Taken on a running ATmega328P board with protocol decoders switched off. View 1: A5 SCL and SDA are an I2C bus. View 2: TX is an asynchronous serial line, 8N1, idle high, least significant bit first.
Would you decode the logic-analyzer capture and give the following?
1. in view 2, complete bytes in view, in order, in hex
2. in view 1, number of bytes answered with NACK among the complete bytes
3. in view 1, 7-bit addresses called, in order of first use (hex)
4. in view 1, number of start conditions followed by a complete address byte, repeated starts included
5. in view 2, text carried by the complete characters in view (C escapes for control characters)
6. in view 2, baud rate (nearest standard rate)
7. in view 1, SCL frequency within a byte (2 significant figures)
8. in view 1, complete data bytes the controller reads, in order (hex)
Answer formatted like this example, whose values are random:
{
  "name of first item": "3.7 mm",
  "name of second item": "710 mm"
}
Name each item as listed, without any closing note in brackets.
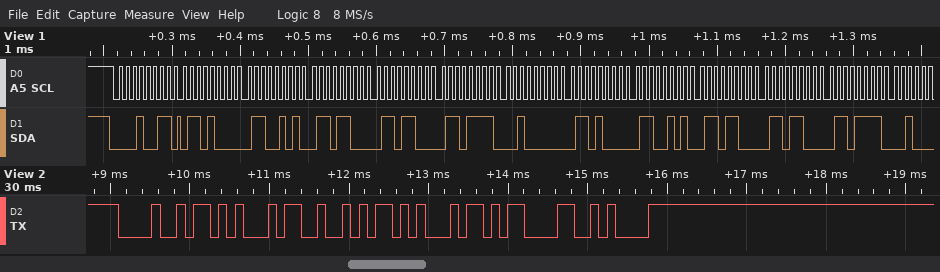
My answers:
{
  "in view 2, complete bytes in view, in order, in hex": "48 45 52 45 0D 0A",
  "in view 1, number of bytes answered with NACK among the complete bytes": "0",
  "in view 1, 7-bit addresses called, in order of first use": "0x09",
  "in view 1, number of start conditions followed by a complete address byte, repeated starts included": "1",
  "in view 2, text carried by the complete characters in view": "\"HERE\\r\\n\"",
  "in view 2, baud rate": "9600 baud",
  "in view 1, SCL frequency within a byte": "100 kHz",
  "in view 1, complete data bytes the controller reads, in order": "68 65 6C 6C 6F 20 68 65 6C 6C 6F"
}
